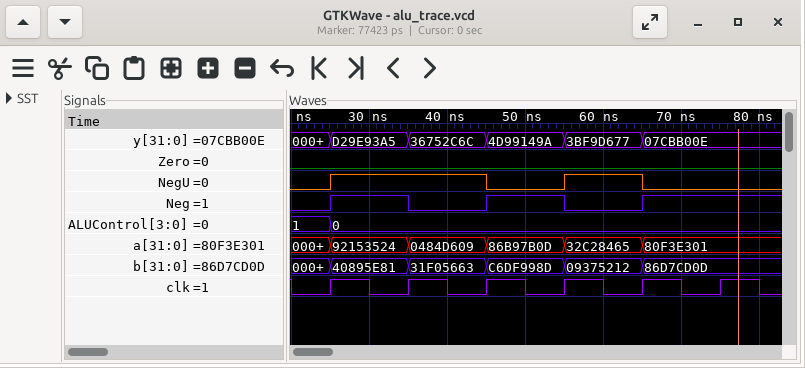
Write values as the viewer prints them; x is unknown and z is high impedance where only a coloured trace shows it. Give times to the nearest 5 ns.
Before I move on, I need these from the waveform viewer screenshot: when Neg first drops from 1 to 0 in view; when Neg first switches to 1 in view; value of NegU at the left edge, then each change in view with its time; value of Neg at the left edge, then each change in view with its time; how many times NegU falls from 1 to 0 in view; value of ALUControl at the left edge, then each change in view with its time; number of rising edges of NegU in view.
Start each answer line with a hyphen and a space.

- 35 ns
- 25 ns
- 0, 1 at 25 ns, 0 at 45 ns, 1 at 55 ns, 0 at 65 ns
- 0, 1 at 25 ns, 0 at 35 ns, 1 at 45 ns, 0 at 55 ns, 1 at 65 ns
- 2
- 1, 0 at 25 ns
- 2
